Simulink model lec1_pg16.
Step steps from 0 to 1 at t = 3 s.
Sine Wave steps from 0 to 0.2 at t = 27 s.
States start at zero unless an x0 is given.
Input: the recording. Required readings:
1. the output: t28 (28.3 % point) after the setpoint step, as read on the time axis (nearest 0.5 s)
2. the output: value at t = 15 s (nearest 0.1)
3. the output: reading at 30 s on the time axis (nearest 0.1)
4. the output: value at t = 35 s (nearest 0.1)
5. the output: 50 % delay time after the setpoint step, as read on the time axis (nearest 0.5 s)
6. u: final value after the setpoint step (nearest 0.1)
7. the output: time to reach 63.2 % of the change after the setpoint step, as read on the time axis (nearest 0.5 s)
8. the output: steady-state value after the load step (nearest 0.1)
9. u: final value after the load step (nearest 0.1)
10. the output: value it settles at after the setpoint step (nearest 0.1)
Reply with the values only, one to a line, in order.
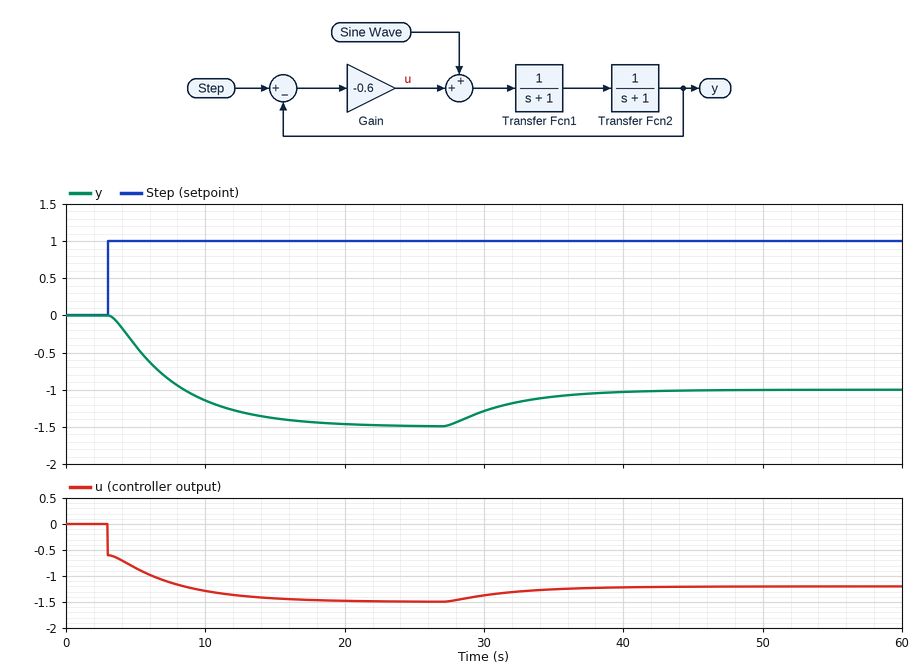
5.0 s
-1.4
-1.3
-1.1
6.5 s
-1.5
8.0 s
-1.0
-1.2
-1.5
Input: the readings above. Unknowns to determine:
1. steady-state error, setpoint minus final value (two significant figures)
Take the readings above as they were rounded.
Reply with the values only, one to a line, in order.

2.5
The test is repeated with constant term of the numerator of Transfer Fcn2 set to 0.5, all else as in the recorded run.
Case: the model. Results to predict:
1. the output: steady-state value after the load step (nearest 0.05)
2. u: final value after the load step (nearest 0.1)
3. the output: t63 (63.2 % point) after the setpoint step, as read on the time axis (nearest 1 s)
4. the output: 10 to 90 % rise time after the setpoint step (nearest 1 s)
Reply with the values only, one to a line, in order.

-0.30
-0.8
6 s
5 s
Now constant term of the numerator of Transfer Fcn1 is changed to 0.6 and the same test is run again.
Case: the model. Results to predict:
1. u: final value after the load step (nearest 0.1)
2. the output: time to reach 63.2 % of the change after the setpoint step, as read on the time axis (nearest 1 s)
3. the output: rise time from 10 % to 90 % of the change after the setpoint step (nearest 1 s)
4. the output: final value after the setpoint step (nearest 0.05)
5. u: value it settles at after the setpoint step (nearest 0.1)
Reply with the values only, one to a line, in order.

-0.8
6 s
6 s
-0.55
-0.9
